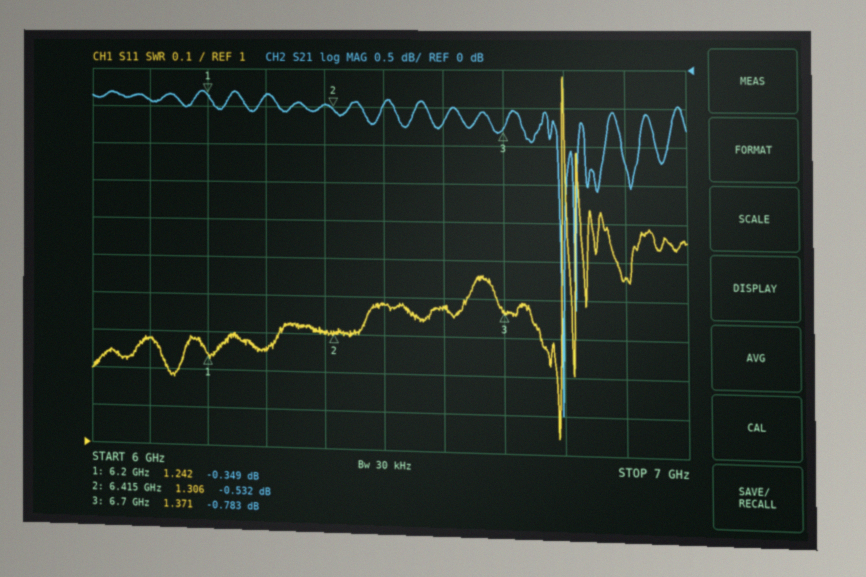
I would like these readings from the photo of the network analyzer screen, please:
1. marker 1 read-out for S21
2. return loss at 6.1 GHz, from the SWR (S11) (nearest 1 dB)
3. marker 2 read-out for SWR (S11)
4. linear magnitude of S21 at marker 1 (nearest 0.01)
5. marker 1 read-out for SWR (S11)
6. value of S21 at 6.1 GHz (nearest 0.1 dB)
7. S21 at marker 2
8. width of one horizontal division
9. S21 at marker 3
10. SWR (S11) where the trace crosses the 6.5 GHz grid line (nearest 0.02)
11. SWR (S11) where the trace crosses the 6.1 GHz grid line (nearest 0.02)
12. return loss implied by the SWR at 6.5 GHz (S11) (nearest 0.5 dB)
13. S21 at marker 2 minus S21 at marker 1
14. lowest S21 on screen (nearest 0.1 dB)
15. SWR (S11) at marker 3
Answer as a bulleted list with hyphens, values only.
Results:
- -0.349 dB
- 18 dB
- 1.306
- 0.96
- 1.242
- -0.4 dB
- -0.532 dB
- 100 MHz
- -0.783 dB
- 1.38
- 1.28
- 16.0 dB
- -0.183 dB
- -4.5 dB
- 1.371
